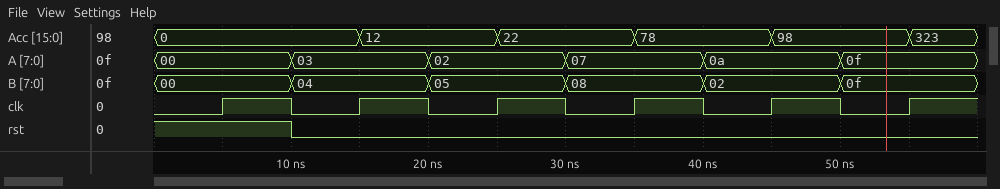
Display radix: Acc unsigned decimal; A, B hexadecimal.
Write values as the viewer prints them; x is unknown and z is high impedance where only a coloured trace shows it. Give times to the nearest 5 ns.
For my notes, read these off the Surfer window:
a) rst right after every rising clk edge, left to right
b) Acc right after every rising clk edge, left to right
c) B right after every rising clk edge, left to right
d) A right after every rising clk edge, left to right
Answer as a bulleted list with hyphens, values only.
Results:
- 1 0 0 0 0 0
- 0, 12, 22, 78, 98, 323
- 00, 04, 05, 08, 02, 0f
- 00, 03, 02, 07, 0a, 0f
